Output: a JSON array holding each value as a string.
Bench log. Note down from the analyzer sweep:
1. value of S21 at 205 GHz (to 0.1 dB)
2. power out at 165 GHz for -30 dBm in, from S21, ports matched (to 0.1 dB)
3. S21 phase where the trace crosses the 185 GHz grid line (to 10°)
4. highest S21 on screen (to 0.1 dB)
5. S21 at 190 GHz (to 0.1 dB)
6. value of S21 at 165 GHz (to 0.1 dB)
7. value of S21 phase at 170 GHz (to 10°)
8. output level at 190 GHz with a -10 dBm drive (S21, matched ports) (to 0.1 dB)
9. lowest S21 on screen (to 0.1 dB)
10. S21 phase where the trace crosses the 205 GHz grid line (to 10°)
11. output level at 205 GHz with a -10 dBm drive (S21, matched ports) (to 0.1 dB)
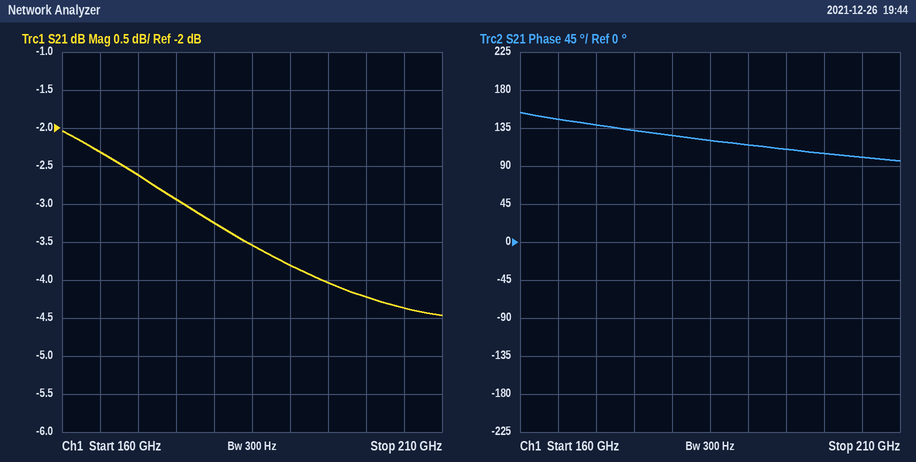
["-4.4 dB", "-32.3 dBm", "120°", "-2.0 dB", "-3.8 dB", "-2.3 dB", "140°", "-13.8 dBm", "-4.5 dB", "100°", "-14.4 dBm"]
